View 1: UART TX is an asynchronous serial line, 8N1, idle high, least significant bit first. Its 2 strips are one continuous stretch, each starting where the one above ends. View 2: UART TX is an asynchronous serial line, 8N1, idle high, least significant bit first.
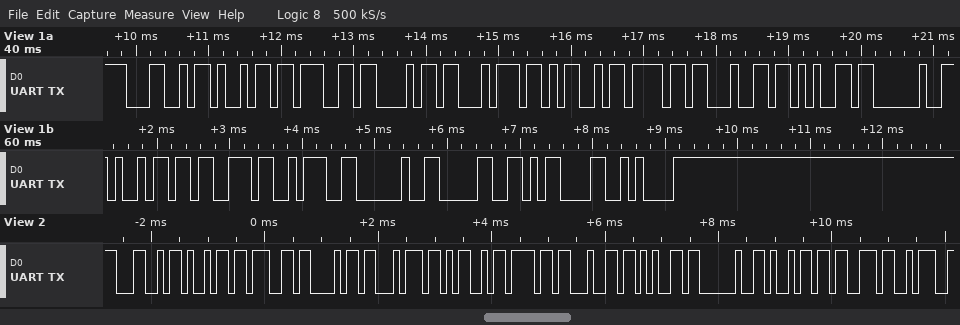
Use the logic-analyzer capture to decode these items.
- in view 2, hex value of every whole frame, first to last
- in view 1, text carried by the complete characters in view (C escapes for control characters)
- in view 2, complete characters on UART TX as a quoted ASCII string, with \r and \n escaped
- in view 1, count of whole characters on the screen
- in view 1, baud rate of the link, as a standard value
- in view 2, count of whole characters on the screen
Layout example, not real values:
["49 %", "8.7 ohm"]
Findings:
["4C 69 67 68 74 4D 6F 64 65 20 69 73 3A", "\"LightMode is: 0\\r\\n\"", "\"LightMode is:\"", "17", "9600 baud", "13"]
